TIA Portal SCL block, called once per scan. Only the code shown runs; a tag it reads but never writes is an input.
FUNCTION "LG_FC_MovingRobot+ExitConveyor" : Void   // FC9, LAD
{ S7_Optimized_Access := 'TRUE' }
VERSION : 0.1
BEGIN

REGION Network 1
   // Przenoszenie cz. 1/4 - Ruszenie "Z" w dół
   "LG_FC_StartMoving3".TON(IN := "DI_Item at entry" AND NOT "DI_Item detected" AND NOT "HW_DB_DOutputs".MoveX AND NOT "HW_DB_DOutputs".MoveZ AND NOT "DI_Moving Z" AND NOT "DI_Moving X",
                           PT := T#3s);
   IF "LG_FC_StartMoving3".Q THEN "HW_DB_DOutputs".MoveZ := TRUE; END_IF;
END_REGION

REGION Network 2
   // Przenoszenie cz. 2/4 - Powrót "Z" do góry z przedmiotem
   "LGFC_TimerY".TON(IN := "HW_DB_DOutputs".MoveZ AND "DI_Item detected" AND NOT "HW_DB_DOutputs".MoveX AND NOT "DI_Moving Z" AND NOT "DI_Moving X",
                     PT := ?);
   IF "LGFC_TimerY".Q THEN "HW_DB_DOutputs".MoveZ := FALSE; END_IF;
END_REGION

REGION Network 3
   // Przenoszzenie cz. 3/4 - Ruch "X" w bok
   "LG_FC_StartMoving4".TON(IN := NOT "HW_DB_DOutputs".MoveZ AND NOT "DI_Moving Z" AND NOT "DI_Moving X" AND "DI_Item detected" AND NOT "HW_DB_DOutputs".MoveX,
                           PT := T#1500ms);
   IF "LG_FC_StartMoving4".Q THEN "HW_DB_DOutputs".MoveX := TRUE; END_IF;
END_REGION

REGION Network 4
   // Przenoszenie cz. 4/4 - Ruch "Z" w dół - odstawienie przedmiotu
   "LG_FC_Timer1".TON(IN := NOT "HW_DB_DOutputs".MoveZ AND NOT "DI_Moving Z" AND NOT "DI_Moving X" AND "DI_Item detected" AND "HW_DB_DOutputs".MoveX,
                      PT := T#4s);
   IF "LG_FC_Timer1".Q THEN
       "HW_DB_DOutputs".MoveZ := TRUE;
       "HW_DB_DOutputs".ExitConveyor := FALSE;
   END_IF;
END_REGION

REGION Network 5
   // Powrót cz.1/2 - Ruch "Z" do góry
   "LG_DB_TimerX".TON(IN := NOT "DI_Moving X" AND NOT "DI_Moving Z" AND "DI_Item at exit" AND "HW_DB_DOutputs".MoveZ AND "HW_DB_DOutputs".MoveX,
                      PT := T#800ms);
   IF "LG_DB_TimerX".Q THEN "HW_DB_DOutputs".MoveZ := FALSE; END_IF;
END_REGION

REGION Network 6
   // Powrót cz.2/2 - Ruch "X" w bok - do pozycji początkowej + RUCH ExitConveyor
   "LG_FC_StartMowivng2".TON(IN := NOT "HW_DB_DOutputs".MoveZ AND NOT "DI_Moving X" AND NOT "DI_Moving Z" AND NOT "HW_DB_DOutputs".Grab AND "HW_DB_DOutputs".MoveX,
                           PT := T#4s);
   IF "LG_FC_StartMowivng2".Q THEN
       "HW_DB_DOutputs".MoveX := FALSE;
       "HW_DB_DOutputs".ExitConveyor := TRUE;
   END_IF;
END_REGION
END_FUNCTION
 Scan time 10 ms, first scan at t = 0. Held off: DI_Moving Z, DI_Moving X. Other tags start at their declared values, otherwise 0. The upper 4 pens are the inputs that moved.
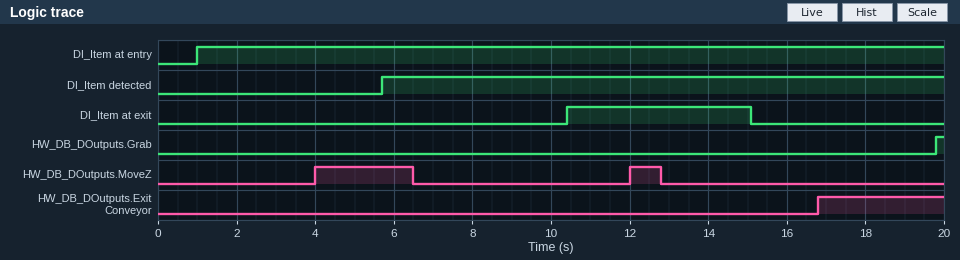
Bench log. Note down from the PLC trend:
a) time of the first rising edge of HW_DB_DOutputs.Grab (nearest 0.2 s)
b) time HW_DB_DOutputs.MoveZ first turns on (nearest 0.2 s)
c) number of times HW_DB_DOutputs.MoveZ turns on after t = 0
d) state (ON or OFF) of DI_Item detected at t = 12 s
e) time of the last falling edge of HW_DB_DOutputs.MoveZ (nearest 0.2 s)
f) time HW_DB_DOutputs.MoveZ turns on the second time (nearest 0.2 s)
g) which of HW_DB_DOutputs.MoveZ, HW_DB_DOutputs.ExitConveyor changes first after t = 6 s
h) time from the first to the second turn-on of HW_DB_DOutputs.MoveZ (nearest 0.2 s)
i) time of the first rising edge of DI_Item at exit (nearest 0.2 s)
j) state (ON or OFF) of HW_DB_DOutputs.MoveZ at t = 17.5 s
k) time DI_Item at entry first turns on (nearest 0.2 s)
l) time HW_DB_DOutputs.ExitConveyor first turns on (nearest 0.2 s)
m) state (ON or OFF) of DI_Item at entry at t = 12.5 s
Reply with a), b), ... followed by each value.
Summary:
a) 19.8 s
b) 4.0 s
c) 2
d) ON
e) 12.8 s
f) 12.0 s
g) HW_DB_DOutputs.MoveZ
h) 8.0 s
i) 10.4 s
j) OFF
k) 1.0 s
l) 16.8 s
m) ON
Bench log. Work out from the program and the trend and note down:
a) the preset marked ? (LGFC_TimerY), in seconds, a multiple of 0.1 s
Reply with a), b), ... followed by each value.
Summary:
a) 0.8 s
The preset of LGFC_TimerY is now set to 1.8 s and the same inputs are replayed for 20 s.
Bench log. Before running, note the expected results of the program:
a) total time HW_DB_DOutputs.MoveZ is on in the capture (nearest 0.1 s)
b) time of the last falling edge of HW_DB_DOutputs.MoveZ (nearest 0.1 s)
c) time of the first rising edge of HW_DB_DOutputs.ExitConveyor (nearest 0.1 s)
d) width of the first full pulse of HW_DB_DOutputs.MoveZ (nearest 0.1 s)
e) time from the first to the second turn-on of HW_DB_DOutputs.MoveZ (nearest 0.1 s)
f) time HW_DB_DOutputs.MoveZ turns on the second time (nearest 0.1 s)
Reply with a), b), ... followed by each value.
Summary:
a) 4.3 s
b) 13.8 s
c) 17.8 s
d) 3.5 s
e) 9.0 s
f) 13.0 s
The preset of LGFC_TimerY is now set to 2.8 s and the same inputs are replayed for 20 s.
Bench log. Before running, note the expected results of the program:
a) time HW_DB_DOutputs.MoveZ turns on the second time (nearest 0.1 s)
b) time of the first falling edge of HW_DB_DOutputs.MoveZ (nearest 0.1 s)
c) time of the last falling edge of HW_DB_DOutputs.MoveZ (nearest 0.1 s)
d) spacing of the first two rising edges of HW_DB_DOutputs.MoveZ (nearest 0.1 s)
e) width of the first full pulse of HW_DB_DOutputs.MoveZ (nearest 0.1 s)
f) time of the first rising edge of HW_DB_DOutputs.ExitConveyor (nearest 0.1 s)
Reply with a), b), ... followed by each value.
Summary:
a) 14.0 s
b) 8.5 s
c) 14.8 s
d) 10.0 s
e) 4.5 s
f) 18.8 s
